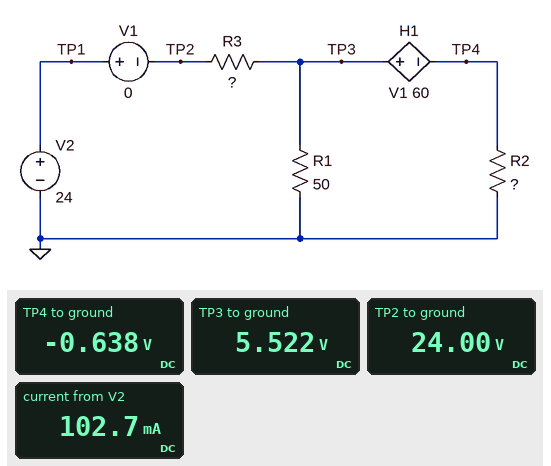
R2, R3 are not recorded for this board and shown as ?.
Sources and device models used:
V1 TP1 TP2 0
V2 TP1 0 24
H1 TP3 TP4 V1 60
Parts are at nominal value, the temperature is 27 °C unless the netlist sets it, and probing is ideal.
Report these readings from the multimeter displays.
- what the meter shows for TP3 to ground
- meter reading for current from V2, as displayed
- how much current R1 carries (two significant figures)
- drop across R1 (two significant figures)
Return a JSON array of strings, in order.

["5.522 V", "102.7 mA", "110 mA", "5.5 V"]
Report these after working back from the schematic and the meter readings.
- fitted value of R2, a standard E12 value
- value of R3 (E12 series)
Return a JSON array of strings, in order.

["82 Ω", "180 Ω"]
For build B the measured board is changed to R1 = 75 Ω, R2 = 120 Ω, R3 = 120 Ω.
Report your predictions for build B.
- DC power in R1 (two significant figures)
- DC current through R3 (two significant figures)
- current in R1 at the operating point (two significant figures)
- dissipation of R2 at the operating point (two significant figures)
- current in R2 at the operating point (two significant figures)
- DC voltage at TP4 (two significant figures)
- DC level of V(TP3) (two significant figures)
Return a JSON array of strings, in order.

["1.0 W", "130 mA", "120 mA", "11 mW", "9.8 mA", "1.2 V", "8.8 V"]
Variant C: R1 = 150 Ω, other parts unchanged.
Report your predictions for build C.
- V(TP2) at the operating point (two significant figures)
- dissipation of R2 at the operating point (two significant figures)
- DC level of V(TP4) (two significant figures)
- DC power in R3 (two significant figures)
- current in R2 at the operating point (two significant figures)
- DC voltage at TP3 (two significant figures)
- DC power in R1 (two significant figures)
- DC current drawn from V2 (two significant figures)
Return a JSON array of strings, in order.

["24 V", "96 mW", "2.8 V", "1.4 W", "34 mA", "8.1 V", "440 mW", "88 mA"]
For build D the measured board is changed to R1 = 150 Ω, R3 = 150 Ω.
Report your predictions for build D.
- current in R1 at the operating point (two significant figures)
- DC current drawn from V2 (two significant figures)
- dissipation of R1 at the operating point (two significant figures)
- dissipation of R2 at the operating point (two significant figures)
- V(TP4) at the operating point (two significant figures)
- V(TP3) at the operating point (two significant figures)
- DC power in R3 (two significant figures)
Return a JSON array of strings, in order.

["61 mA", "99 mA", "550 mW", "120 mW", "3.2 V", "9.1 V", "1.5 W"]
